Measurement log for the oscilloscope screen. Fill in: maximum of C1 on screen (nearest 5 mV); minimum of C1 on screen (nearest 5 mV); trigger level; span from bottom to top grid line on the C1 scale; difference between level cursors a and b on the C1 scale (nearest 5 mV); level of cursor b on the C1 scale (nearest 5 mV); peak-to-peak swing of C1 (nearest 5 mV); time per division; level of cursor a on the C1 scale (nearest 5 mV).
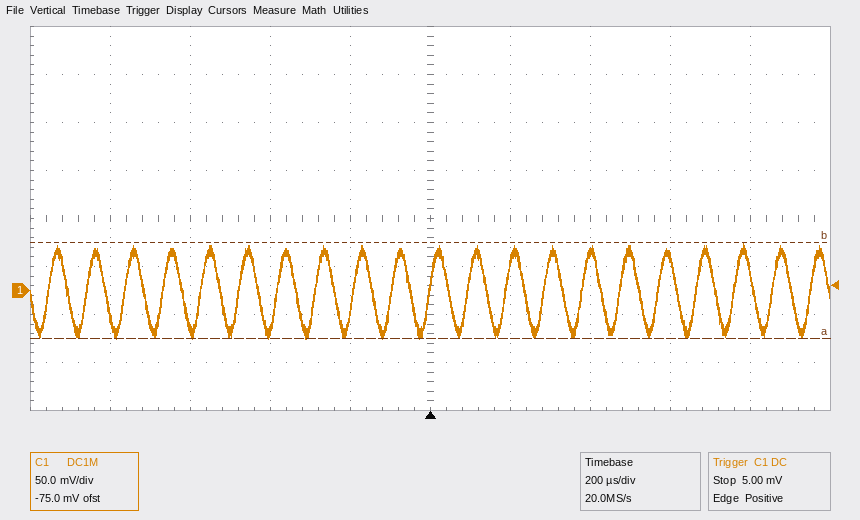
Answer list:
50 mV
-50 mV
5.00 mV
400 mV
100 mV
50 mV
100 mV
200 µs
-50 mV
